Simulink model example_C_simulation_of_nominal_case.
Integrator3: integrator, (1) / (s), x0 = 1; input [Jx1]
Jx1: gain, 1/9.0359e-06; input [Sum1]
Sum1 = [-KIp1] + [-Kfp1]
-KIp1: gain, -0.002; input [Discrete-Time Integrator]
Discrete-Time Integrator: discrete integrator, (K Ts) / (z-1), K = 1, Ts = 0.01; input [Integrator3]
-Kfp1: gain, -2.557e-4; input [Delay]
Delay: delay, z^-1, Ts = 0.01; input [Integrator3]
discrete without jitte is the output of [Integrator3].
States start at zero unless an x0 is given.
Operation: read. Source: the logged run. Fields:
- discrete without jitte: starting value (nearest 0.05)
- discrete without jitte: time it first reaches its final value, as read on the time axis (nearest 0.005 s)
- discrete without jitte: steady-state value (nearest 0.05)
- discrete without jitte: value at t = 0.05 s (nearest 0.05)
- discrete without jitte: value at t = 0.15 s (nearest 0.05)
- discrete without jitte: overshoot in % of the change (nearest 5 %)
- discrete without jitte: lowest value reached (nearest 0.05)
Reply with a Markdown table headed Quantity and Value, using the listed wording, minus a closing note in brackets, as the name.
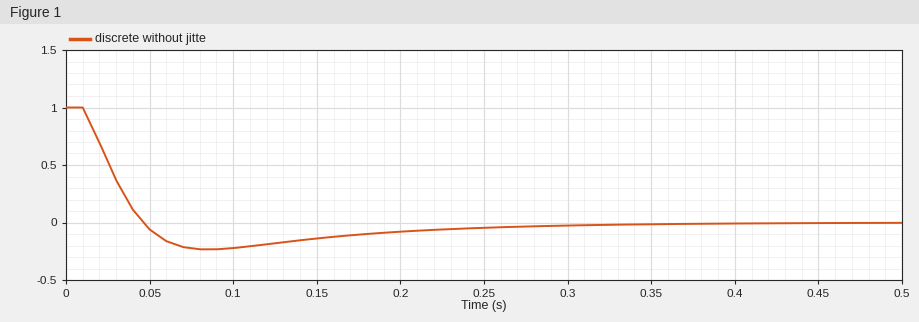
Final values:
| Quantity | Value |
|---|---|
| discrete without jitte: starting value | 1.00 |
| discrete without jitte: time it first reaches its final value, as read on the time axis | 0.045 s |
| discrete without jitte: steady-state value | 0.00 |
| discrete without jitte: value at t = 0.05 s | -0.05 |
| discrete without jitte: value at t = 0.15 s | -0.15 |
| discrete without jitte: overshoot in % of the change | 25 % |
| discrete without jitte: lowest value reached | -0.25 |
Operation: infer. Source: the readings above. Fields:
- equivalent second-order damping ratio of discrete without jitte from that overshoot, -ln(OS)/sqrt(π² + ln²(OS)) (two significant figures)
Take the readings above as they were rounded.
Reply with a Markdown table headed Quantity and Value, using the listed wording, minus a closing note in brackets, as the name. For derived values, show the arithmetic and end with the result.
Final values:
| Quantity | Value |
|---|---|
| equivalent second-order damping ratio of discrete without jitte from that overshoot, -ln(OS)/sqrt(π² + ln²(OS)) | ln(0.25) = -1.386; 1.386 / sqrt(9.870 + 1.922) = 0.40 |
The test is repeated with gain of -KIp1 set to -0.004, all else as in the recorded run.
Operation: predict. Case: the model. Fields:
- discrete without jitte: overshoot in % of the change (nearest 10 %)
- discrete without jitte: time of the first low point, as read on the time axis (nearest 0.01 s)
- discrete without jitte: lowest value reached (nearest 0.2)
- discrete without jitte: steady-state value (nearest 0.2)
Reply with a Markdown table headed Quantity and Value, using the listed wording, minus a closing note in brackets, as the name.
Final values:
| Quantity | Value |
|---|---|
| discrete without jitte: overshoot in % of the change | 40 % |
| discrete without jitte: time of the first low point, as read on the time axis | 0.08 s |
| discrete without jitte: lowest value reached | -0.4 |
| discrete without jitte: steady-state value | 0.0 |
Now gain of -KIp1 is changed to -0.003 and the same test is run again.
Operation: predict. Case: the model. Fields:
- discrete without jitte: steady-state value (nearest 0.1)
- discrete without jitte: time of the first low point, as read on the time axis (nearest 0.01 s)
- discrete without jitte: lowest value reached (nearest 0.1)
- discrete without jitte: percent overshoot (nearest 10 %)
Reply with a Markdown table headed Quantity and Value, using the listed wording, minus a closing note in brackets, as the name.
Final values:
| Quantity | Value |
|---|---|
| discrete without jitte: steady-state value | 0.0 |
| discrete without jitte: time of the first low point, as read on the time axis | 0.08 s |
| discrete without jitte: lowest value reached | -0.3 |
| discrete without jitte: percent overshoot | 30 % |
